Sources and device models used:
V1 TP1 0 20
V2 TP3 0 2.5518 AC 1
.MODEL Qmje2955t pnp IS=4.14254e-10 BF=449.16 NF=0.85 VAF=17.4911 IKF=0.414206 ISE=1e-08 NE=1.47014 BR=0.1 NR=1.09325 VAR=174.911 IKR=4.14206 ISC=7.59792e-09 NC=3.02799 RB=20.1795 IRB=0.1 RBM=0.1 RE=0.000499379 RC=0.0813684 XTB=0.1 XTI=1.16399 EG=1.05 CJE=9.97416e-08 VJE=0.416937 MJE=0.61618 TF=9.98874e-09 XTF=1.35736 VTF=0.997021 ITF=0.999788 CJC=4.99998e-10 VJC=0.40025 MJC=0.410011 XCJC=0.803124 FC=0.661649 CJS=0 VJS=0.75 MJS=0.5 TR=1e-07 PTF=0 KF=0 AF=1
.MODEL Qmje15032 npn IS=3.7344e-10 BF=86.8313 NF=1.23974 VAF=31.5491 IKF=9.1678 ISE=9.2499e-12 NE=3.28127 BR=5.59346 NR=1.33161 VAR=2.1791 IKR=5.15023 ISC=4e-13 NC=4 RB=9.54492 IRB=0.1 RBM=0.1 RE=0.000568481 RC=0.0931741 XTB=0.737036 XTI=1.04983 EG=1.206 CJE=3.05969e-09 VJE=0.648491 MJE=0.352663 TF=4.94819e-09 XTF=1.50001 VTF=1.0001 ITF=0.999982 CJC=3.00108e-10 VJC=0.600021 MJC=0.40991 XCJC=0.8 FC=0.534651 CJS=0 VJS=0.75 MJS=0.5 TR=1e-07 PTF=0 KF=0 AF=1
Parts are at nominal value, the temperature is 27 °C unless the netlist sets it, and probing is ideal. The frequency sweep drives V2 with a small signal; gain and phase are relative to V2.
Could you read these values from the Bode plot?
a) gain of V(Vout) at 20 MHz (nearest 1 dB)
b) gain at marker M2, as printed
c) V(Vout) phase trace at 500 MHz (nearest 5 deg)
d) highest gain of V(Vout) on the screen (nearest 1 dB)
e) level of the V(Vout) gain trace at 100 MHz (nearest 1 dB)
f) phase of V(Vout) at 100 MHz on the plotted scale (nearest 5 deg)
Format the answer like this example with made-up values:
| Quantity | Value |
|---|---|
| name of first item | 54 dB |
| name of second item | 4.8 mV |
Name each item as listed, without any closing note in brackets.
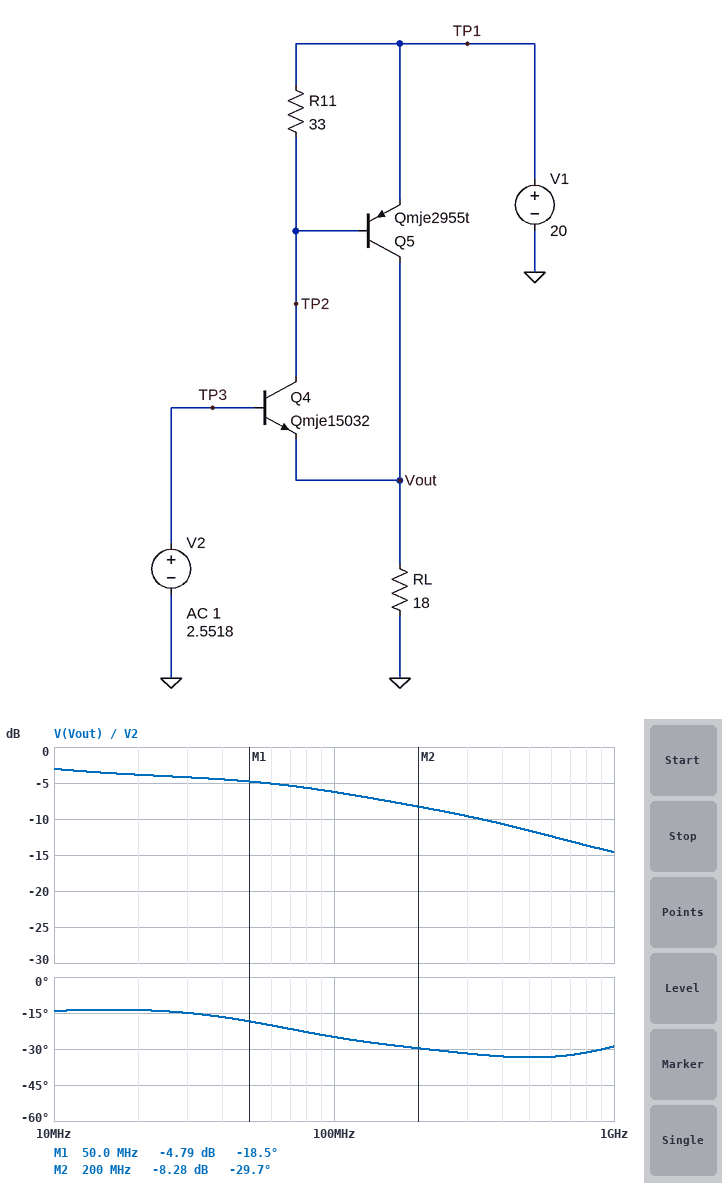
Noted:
| Quantity | Value |
|---|---|
| gain of V(Vout) at 20 MHz | -4 dB |
| gain at marker M2, as printed | -8.28 dB |
| V(Vout) phase trace at 500 MHz | -35 deg |
| highest gain of V(Vout) on the screen | -3 dB |
| level of the V(Vout) gain trace at 100 MHz | -6 dB |
| phase of V(Vout) at 100 MHz on the plotted scale | -25 deg |
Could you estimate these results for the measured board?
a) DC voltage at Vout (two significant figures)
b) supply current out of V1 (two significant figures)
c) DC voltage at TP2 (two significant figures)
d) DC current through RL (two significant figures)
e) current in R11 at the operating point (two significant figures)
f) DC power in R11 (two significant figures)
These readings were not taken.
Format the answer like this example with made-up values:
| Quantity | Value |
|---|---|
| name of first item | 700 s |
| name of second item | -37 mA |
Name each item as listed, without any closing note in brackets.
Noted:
| Quantity | Value |
|---|---|
| DC voltage at Vout | 2.0 V |
| supply current out of V1 | 110 mA |
| DC voltage at TP2 | 20 V |
| DC current through RL | 110 mA |
| current in R11 at the operating point | 13 mA |
| DC power in R11 | 5.4 mW |
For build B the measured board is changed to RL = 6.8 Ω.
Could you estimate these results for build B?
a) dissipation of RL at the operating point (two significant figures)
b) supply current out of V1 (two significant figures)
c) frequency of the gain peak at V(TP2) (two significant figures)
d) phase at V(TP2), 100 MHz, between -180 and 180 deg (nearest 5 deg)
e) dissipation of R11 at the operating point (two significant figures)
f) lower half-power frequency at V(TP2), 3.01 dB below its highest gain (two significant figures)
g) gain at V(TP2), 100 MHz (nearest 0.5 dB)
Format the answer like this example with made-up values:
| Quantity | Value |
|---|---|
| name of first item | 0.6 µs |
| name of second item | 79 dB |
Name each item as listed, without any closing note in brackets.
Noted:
| Quantity | Value |
|---|---|
| dissipation of RL at the operating point | 590 mW |
| supply current out of V1 | 290 mA |
| frequency of the gain peak at V(TP2) | 3.1 MHz |
| phase at V(TP2), 100 MHz, between -180 and 180 deg | 45 deg |
| dissipation of R11 at the operating point | 6.6 mW |
| lower half-power frequency at V(TP2), 3.01 dB below its highest gain | 1.4 MHz |
| gain at V(TP2), 100 MHz | -10.0 dB |
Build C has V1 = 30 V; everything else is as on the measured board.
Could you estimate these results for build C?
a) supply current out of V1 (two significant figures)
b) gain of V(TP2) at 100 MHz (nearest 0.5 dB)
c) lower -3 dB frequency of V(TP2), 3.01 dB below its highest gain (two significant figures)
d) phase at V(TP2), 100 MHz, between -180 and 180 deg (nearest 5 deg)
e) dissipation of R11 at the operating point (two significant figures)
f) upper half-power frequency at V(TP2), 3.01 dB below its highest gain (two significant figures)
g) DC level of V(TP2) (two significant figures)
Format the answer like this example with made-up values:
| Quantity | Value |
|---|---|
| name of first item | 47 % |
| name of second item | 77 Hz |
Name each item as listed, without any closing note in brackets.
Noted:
| Quantity | Value |
|---|---|
| supply current out of V1 | 110 mA |
| gain of V(TP2) at 100 MHz | -9.5 dB |
| lower -3 dB frequency of V(TP2), 3.01 dB below its highest gain | 930 kHz |
| phase at V(TP2), 100 MHz, between -180 and 180 deg | 45 deg |
| dissipation of R11 at the operating point | 5.2 mW |
| upper half-power frequency at V(TP2), 3.01 dB below its highest gain | 8.5 MHz |
| DC level of V(TP2) | 30 V |
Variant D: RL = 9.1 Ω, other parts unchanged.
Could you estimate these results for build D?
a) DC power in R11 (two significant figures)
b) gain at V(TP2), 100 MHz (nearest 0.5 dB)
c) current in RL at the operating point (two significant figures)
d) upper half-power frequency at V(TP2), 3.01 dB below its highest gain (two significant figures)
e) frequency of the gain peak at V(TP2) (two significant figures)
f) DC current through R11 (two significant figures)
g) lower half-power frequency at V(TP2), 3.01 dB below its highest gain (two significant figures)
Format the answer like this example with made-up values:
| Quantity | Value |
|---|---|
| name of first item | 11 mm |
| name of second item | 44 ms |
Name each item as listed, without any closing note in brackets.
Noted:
| Quantity | Value |
|---|---|
| DC power in R11 | 6.2 mW |
| gain at V(TP2), 100 MHz | -9.5 dB |
| current in RL at the operating point | 220 mA |
| upper half-power frequency at V(TP2), 3.01 dB below its highest gain | 7.4 MHz |
| frequency of the gain peak at V(TP2) | 3.0 MHz |
| DC current through R11 | 14 mA |
| lower half-power frequency at V(TP2), 3.01 dB below its highest gain | 1.3 MHz |
